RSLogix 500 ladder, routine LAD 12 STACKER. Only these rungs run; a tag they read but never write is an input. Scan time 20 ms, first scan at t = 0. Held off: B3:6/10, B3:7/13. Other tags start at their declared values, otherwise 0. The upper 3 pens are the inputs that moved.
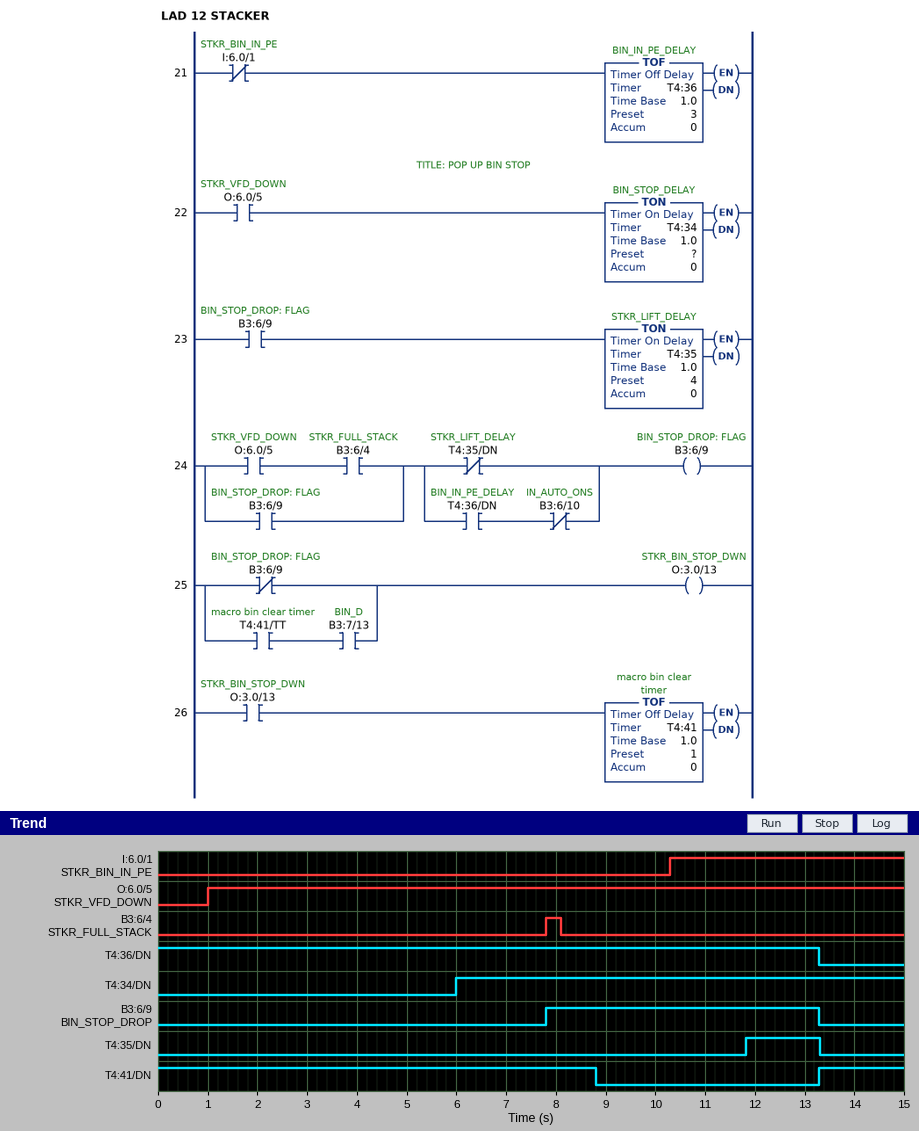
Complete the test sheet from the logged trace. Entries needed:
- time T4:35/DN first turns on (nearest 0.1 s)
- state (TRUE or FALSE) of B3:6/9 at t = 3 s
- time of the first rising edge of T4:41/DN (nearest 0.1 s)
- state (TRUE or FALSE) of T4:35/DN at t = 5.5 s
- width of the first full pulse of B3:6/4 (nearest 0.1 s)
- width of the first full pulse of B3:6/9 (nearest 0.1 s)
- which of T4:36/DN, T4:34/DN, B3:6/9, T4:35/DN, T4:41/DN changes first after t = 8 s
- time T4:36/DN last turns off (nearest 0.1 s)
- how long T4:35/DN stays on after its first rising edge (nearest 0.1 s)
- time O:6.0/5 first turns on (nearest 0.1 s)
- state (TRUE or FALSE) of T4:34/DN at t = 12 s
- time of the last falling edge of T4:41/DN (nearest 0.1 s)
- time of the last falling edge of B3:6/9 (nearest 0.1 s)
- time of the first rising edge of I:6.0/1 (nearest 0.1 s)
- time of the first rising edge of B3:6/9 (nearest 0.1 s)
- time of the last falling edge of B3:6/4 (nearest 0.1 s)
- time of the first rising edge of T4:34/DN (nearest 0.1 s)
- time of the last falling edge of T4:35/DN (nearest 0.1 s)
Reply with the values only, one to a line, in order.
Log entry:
11.8 s
FALSE
13.3 s
FALSE
0.3 s
5.5 s
T4:41/DN
13.3 s
1.5 s
1.0 s
TRUE
8.8 s
13.3 s
10.3 s
7.8 s
8.1 s
6.0 s
13.3 s
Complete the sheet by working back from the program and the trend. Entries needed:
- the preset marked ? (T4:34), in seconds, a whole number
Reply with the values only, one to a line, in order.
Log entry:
5 s
